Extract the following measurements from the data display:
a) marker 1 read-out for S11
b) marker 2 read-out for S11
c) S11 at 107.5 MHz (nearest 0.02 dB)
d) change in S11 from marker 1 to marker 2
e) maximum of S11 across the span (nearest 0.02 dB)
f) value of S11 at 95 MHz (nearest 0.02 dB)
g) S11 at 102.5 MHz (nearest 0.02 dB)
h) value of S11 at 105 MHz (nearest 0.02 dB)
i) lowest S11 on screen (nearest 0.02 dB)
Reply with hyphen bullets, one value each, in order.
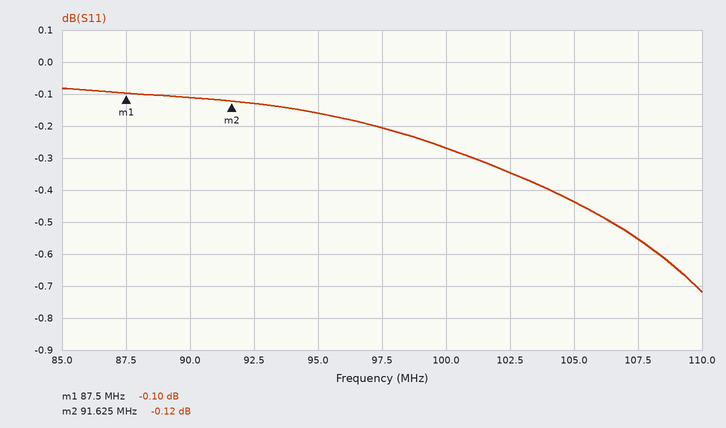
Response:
- -0.10 dB
- -0.12 dB
- -0.56 dB
- -0.02 dB
- -0.08 dB
- -0.16 dB
- -0.34 dB
- -0.44 dB
- -0.72 dB
